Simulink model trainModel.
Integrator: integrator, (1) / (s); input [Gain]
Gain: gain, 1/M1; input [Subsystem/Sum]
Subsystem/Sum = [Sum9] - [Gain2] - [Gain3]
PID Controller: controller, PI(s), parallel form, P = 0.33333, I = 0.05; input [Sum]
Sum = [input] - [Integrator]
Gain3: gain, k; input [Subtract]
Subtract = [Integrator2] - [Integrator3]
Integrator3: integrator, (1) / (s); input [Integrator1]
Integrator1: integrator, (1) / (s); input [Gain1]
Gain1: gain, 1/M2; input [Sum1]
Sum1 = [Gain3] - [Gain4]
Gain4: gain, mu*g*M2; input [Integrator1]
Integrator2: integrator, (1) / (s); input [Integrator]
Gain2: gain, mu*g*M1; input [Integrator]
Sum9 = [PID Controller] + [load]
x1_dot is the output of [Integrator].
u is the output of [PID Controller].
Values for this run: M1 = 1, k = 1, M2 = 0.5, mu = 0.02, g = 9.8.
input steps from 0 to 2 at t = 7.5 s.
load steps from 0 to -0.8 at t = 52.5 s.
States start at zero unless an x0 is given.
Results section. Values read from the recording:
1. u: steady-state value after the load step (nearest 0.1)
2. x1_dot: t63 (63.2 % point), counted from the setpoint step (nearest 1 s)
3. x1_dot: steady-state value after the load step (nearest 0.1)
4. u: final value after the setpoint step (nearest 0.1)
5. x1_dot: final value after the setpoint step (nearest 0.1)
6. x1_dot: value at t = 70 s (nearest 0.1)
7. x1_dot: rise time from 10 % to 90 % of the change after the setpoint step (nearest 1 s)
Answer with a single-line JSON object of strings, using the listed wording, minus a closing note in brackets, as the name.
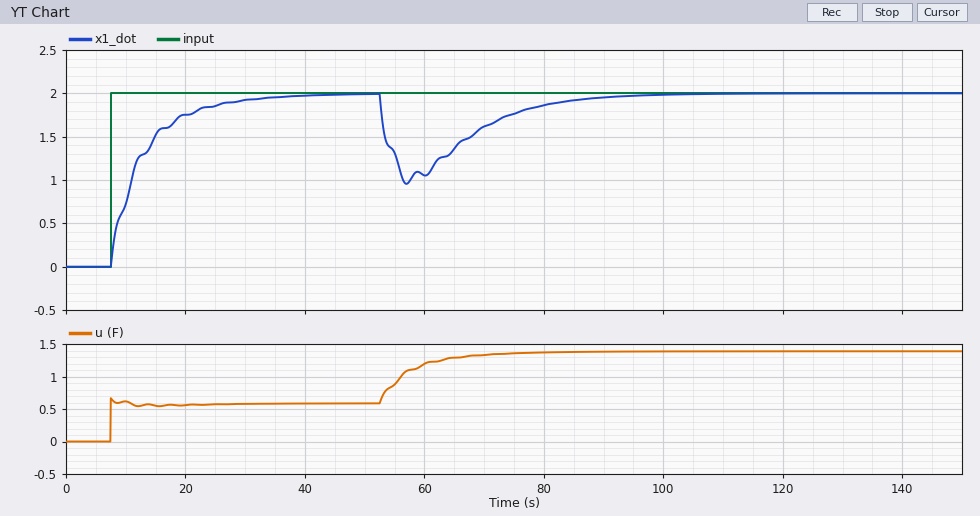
{"u: steady-state value after the load step": "1.4", "x1_dot: t63 (63.2 % point), counted from the setpoint step": "5 s", "x1_dot: steady-state value after the load step": "2.0", "u: final value after the setpoint step": "0.6", "x1_dot: final value after the setpoint step": "2.0", "x1_dot: value at t = 70 s": "1.6", "x1_dot: rise time from 10 % to 90 % of the change after the setpoint step": "14 s"}
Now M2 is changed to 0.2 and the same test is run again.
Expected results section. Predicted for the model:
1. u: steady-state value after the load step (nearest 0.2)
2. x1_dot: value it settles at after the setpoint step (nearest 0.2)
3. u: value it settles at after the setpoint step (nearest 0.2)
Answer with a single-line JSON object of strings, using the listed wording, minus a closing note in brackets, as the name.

{"u: steady-state value after the load step": "1.2", "x1_dot: value it settles at after the setpoint step": "2.0", "u: value it settles at after the setpoint step": "0.4"}
